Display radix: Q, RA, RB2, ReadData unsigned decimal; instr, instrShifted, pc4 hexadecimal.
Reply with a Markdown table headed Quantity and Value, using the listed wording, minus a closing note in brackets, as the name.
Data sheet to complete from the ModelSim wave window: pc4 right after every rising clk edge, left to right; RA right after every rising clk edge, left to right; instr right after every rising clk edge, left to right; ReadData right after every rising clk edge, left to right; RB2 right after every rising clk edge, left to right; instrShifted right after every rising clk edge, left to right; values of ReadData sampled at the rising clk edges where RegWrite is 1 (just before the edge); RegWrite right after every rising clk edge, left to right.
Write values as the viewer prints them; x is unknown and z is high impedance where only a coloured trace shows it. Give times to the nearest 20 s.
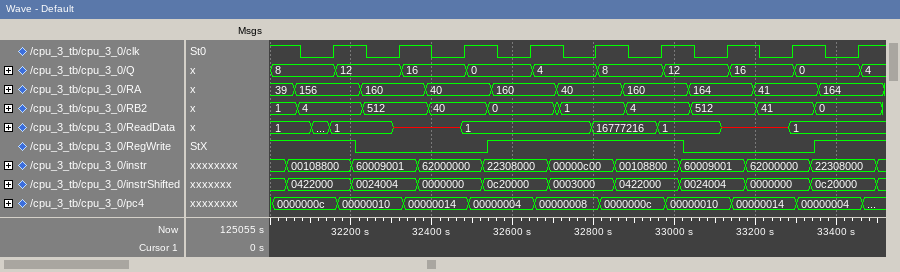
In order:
| Quantity | Value |
|---|---|
| pc4 right after every rising clk edge, left to right | 0000000c, 00000010, 00000014, 00000004, 00000008, 0000000c, 00000010, 00000014, 00000004 |
| RA right after every rising clk edge, left to right | 156, 160, 40, 160, 40, 160, 164, 41, 164 |
| instr right after every rising clk edge, left to right | 00108800, 60009001, 62000000, 22308000, 00000c00, 00108800, 60009001, 62000000, 22308000 |
| ReadData right after every rising clk edge, left to right | 1, x, 1, 1, 16777216, 1, x, 1, 1 |
| RB2 right after every rising clk edge, left to right | 4, 512, 40, 0, 1, 4, 512, 41, 0 |
| instrShifted right after every rising clk edge, left to right | 0422000, 0024004, 0000000, 0c20000, 0003000, 0422000, 0024004, 0000000, 0c20000 |
| values of ReadData sampled at the rising clk edges where RegWrite is 1 | 1, 1, 16777216, 1, 1 |
| RegWrite right after every rising clk edge, left to right | 1 0 0 1 1 1 0 0 1 |
